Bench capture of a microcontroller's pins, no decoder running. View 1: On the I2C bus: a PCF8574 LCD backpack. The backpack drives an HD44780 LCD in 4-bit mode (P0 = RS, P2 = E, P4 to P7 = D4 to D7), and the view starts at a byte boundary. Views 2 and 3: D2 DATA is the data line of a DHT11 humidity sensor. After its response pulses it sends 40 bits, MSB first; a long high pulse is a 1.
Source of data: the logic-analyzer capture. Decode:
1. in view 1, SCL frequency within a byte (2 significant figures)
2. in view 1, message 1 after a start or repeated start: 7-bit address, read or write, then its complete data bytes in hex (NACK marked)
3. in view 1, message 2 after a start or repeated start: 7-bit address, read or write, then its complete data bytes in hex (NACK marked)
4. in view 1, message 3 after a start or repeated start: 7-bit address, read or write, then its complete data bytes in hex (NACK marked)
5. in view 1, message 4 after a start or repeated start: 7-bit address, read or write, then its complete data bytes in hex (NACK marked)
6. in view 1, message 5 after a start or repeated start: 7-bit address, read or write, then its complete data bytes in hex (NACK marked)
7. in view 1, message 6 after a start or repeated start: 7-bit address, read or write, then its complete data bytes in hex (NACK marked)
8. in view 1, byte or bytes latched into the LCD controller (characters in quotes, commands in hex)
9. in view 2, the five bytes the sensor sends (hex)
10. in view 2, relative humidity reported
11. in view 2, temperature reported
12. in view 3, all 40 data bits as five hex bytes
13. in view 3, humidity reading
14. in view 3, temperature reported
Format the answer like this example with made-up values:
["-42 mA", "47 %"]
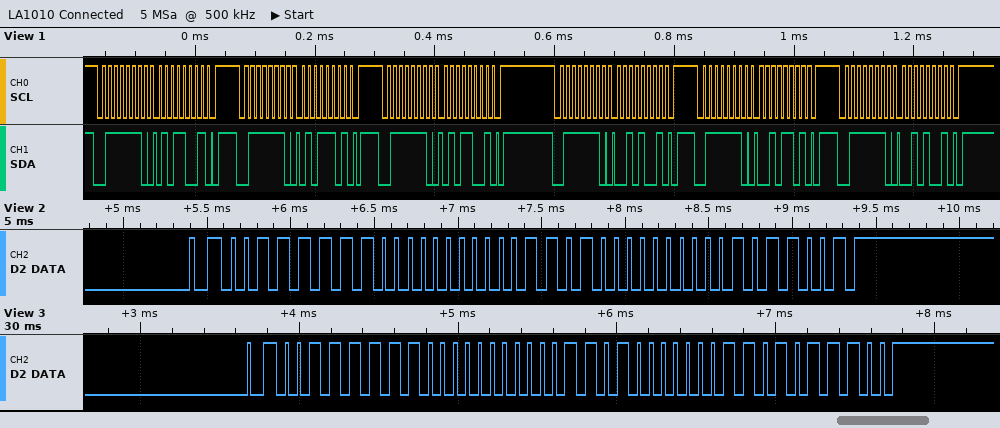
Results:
["100 kHz", "0x3F write: 59", "0x3F write: 5D", "0x3F write: 59", "0x3F write: 29", "0x3F write: 2D", "0x3F write: 29", "'R'", "3F 00 1A 00 59", "63 %", "26.0 °C", "3F 00 1A 03 5C", "63 %", "26.3 °C"]
